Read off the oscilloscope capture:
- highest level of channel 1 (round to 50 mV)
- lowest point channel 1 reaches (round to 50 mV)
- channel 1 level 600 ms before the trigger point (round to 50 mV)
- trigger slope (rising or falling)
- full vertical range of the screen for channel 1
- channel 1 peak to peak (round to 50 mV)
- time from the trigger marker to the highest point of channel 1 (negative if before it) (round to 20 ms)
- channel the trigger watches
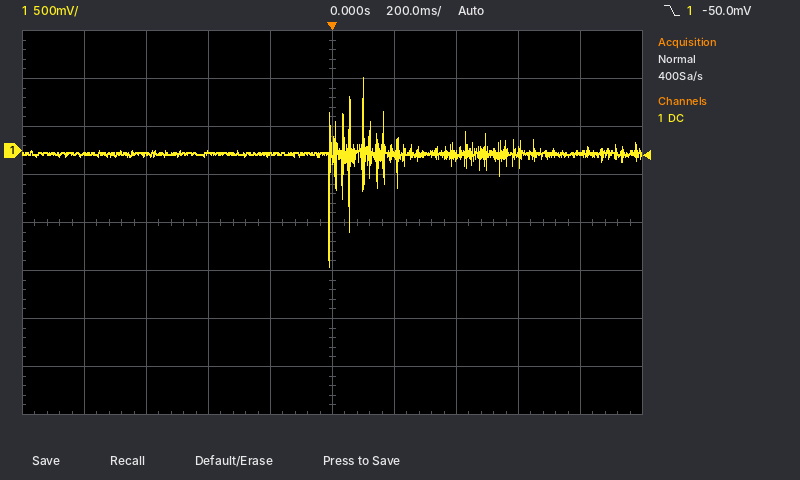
750 mV
-1.20 V
-50 mV
falling
4 V
1.95 V
+100 ms
channel 1
